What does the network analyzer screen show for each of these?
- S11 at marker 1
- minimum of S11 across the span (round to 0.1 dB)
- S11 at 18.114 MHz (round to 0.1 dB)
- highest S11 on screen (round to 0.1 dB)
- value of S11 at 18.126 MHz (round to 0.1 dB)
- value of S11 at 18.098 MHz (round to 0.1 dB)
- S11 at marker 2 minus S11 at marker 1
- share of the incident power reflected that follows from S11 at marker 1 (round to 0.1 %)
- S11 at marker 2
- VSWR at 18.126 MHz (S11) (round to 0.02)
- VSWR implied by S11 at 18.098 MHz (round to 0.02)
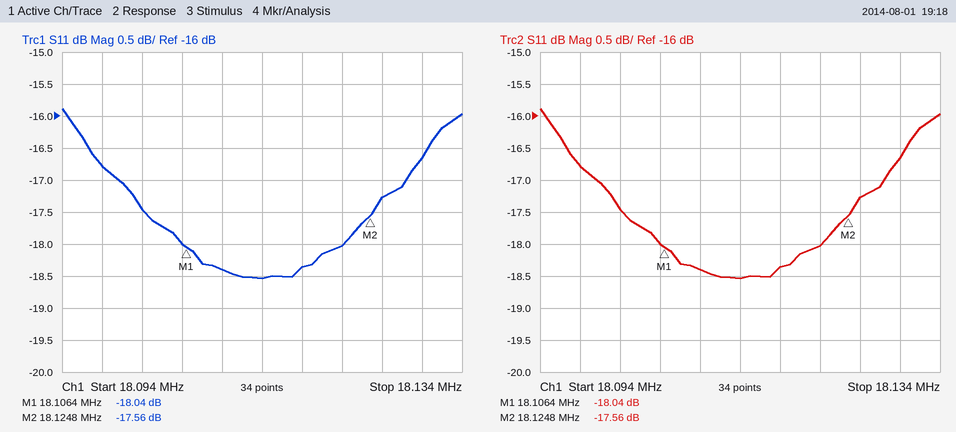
-18.04 dB
-18.5 dB
-18.5 dB
-15.9 dB
-17.3 dB
-16.8 dB
0.48 dB
1.6 %
-17.56 dB
1.32
1.34
